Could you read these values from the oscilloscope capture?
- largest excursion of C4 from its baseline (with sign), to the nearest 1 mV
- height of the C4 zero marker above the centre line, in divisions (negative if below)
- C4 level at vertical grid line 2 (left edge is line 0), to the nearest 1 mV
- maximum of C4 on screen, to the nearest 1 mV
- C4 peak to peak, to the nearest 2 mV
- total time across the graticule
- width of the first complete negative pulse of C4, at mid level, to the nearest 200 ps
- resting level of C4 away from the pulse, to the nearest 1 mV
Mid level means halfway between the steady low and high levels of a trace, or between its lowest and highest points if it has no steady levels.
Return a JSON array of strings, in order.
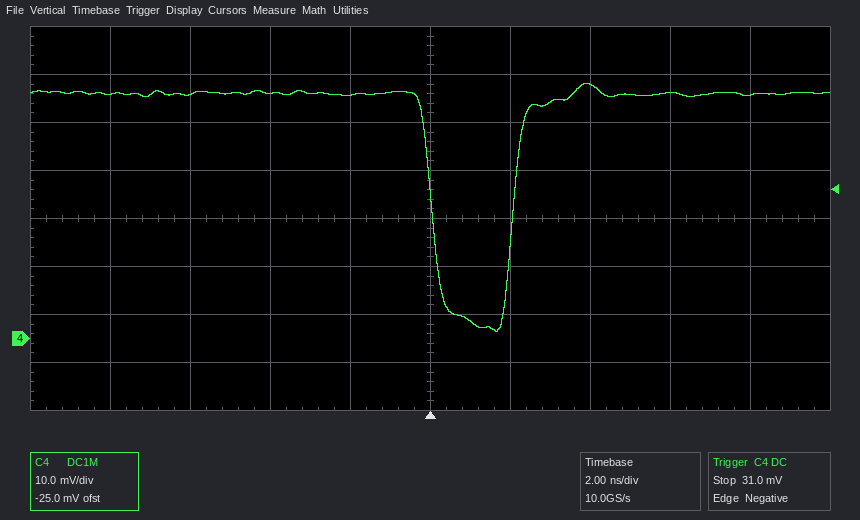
["-50 mV", "-2.5 div", "51 mV", "53 mV", "52 mV", "20 ns", "2.0 ns", "51 mV"]
